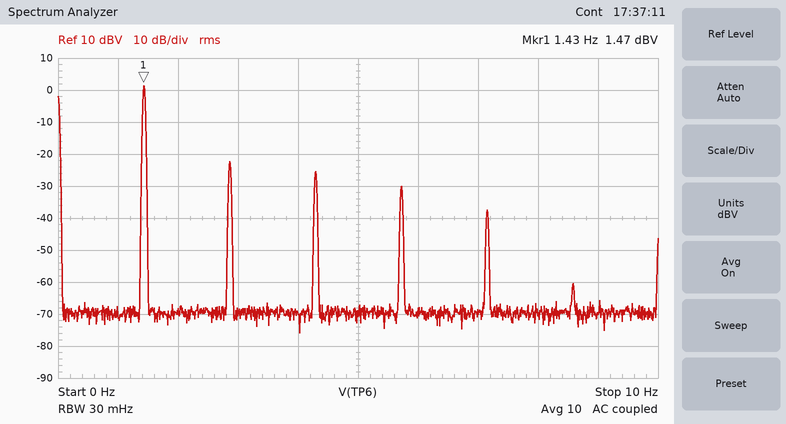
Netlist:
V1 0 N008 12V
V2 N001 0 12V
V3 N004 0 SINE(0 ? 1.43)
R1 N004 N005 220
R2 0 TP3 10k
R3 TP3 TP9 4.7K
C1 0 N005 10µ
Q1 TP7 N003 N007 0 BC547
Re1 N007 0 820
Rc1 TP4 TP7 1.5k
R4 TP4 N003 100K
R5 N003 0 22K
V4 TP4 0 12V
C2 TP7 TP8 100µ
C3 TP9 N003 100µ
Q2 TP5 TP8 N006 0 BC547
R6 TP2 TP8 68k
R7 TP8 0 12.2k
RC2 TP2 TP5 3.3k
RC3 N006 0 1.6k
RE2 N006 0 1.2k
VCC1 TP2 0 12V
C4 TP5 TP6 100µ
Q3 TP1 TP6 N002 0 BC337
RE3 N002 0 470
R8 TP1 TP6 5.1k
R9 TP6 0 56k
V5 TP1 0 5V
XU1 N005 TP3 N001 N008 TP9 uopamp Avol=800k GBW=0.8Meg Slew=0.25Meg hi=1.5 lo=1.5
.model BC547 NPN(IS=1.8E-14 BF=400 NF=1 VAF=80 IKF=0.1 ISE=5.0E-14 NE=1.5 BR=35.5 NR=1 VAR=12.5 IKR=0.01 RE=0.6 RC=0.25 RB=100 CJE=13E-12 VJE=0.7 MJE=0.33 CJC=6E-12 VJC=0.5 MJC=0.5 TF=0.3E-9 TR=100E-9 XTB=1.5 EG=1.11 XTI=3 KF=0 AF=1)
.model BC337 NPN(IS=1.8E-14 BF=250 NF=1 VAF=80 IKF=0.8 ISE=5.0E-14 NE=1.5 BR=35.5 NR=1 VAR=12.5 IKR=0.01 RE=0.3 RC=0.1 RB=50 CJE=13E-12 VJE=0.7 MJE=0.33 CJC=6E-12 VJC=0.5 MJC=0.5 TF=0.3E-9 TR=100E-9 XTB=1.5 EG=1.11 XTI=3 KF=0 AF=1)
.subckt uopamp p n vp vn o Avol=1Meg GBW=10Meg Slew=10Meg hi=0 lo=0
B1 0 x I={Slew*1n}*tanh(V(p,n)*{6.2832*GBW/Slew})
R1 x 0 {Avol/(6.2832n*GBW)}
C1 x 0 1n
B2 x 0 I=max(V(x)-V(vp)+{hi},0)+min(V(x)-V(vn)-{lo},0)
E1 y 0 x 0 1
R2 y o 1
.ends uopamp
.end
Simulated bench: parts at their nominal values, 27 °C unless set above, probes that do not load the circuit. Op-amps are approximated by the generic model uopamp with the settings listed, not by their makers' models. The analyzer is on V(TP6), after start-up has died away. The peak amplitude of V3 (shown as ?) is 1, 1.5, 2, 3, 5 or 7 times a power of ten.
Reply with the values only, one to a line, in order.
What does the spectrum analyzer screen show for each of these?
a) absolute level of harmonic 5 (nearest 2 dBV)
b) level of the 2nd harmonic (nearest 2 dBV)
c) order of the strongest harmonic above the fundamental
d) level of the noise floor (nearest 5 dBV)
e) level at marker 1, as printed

-38 dBV
-22 dBV
2
-70 dBV
1.47 dBV
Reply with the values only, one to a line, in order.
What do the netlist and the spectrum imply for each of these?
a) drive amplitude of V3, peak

300 mV
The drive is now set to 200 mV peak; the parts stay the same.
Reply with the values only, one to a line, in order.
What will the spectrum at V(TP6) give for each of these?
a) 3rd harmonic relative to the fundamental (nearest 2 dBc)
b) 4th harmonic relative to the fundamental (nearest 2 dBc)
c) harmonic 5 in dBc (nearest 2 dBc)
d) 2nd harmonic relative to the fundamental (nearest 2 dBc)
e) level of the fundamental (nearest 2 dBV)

-56 dBc
-58 dBc
-60 dBc
-50 dBc
-2 dBV
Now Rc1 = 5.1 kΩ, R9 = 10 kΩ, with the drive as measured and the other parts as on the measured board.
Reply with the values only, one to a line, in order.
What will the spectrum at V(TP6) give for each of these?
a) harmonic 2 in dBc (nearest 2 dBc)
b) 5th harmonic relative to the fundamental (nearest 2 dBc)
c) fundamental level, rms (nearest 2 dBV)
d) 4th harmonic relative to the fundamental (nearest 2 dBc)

-18 dBc
-40 dBc
8 dBV
-34 dBc
